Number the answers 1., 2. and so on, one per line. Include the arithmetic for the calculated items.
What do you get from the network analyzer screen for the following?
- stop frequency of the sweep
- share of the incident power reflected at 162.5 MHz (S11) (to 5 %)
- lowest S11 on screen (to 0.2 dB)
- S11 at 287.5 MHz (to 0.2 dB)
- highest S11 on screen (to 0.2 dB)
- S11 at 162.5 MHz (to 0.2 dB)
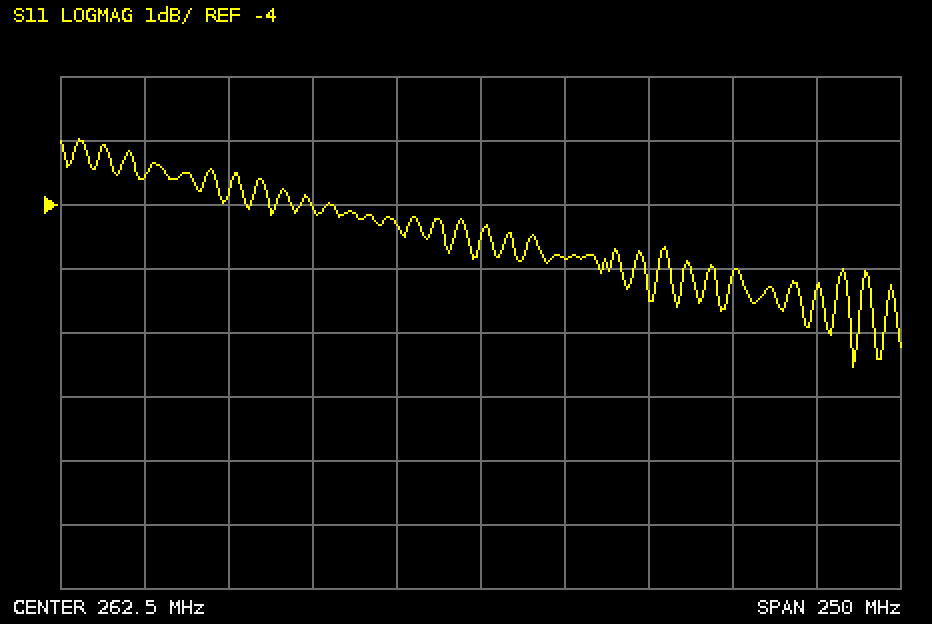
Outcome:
1. 387.5 MHz
2. 10^(-3.6/10) ≈ 43.7 %, so 45 % to the nearest 5 %
3. -6.6 dB
4. -4.8 dB
5. -3.0 dB
6. -3.6 dB
